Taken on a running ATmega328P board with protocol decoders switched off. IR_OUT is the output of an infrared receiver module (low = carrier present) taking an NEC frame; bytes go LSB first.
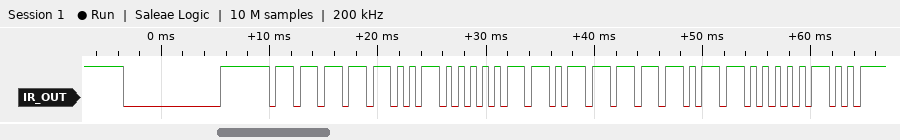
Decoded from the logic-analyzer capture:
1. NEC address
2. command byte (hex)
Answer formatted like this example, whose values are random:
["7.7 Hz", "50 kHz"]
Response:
["0x9F", "0xDF"]
